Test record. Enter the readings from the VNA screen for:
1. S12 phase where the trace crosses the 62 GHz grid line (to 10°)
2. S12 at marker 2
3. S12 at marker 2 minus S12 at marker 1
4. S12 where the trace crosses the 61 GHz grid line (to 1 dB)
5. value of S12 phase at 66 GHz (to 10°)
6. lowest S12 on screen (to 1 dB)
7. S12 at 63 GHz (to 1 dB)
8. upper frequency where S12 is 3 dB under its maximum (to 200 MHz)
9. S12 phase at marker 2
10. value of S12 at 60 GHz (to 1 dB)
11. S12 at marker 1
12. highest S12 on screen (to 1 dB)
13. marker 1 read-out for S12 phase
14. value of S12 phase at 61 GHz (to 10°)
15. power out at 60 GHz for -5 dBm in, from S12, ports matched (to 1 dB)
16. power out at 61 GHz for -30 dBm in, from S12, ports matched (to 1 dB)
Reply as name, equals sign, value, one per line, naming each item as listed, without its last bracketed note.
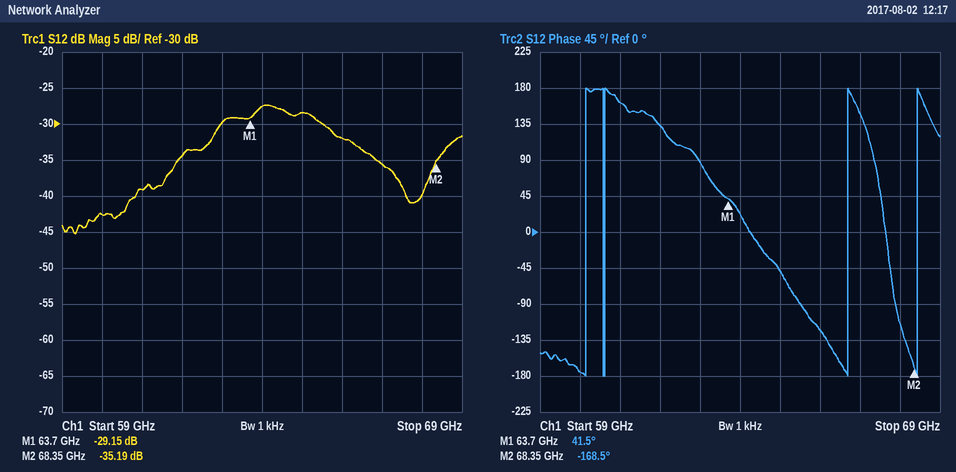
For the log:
S12 phase where the trace crosses the 62 GHz grid line = 130°
S12 at marker 2 = -35.19 dB
S12 at marker 2 minus S12 at marker 1 = -6.04 dB
S12 where the trace crosses the 61 GHz grid line = -39 dB
value of S12 phase at 66 GHz = -120°
lowest S12 on screen = -45 dB
S12 at 63 GHz = -30 dB
upper frequency where S12 is 3 dB under its maximum = 65.6 GHz
S12 phase at marker 2 = -168.5°
value of S12 at 60 GHz = -43 dB
S12 at marker 1 = -29.15 dB
highest S12 on screen = -27 dB
marker 1 read-out for S12 phase = 41.5°
value of S12 phase at 61 GHz = 160°
power out at 60 GHz for -5 dBm in, from S12, ports matched = -48 dBm
power out at 61 GHz for -30 dBm in, from S12, ports matched = -69 dBm
